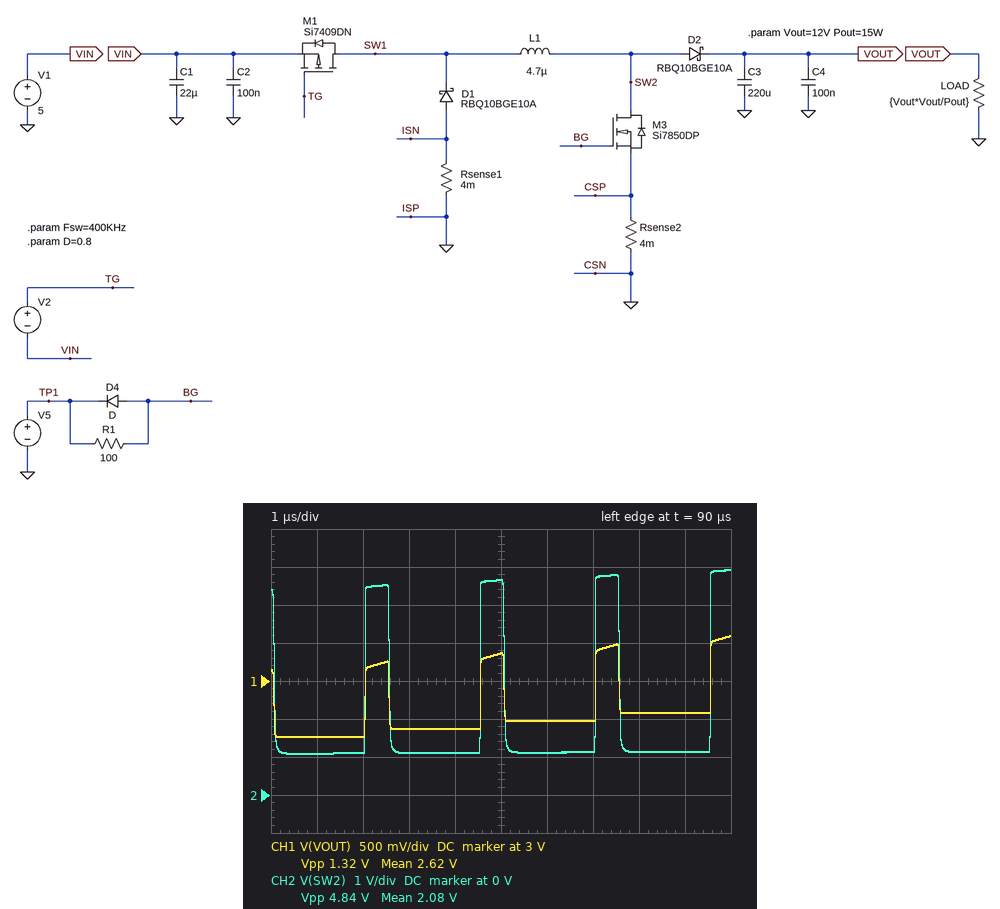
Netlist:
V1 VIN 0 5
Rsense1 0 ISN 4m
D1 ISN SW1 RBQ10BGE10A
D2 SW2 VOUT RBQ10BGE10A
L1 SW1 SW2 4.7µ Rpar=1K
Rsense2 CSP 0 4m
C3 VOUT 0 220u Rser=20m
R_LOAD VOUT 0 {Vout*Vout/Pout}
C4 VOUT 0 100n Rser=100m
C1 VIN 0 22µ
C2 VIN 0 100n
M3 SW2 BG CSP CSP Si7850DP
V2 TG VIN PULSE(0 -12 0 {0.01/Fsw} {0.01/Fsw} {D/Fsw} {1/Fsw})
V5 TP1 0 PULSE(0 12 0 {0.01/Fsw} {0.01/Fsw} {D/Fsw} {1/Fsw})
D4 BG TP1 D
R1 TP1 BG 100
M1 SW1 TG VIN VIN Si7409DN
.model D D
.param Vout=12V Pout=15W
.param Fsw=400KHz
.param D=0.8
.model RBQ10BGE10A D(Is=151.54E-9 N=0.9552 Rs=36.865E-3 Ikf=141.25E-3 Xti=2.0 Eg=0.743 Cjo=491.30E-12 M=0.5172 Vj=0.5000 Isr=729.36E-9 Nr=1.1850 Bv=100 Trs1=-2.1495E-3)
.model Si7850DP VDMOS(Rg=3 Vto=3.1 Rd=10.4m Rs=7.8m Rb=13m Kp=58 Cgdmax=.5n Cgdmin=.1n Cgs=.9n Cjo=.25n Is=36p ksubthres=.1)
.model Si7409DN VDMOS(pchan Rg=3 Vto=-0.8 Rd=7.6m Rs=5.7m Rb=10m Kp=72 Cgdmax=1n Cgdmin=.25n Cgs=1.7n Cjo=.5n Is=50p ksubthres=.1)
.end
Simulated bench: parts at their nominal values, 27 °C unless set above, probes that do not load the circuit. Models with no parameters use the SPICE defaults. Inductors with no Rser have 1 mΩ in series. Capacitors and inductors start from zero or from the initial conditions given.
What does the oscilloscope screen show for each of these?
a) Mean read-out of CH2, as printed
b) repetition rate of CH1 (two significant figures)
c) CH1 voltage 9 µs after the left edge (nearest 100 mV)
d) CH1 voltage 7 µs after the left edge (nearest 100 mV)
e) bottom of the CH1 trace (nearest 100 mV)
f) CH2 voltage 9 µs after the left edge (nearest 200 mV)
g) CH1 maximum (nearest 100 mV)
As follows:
2.08 V
400 kHz
2.6 V
2.5 V
2.3 V
1.2 V
3.6 V
